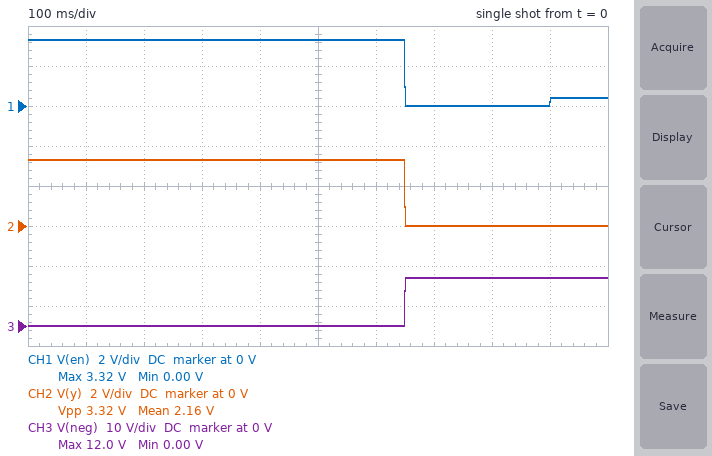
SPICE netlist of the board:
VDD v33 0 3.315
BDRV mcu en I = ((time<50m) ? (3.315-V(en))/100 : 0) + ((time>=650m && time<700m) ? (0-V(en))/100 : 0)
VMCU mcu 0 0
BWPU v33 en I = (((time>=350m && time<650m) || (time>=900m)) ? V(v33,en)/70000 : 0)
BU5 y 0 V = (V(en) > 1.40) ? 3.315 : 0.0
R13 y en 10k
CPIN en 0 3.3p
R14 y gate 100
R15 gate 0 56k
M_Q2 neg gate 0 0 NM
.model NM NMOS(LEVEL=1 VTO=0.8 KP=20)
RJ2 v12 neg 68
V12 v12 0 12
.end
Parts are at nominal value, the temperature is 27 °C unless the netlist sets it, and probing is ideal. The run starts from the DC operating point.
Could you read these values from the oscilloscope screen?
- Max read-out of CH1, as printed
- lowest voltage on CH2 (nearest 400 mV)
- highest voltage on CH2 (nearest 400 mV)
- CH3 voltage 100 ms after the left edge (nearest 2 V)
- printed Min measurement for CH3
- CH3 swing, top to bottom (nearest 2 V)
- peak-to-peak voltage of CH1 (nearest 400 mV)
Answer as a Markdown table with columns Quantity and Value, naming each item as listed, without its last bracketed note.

| Quantity | Value |
|---|---|
| Max read-out of CH1, as printed | 3.32 V |
| lowest voltage on CH2 | 0 V |
| highest voltage on CH2 | 3.2 V |
| CH3 voltage 100 ms after the left edge | 0 V |
| printed Min measurement for CH3 | 0.00 V |
| CH3 swing, top to bottom | 12 V |
| peak-to-peak voltage of CH1 | 3.2 V |
